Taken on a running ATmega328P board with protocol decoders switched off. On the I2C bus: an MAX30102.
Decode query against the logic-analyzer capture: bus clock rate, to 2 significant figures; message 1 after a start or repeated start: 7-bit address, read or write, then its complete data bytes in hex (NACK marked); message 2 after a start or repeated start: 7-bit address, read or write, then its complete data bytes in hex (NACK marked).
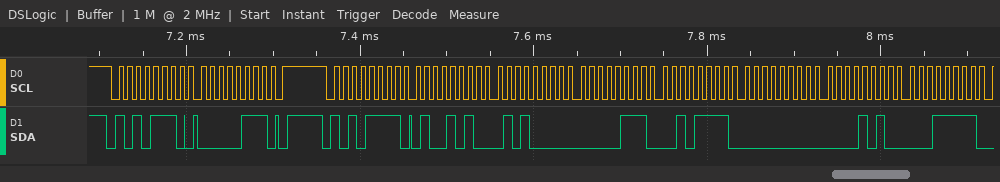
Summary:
100 kHz
0x57 write: 07
0x57 read: 4A 50 07 2F 00 0A 1F
